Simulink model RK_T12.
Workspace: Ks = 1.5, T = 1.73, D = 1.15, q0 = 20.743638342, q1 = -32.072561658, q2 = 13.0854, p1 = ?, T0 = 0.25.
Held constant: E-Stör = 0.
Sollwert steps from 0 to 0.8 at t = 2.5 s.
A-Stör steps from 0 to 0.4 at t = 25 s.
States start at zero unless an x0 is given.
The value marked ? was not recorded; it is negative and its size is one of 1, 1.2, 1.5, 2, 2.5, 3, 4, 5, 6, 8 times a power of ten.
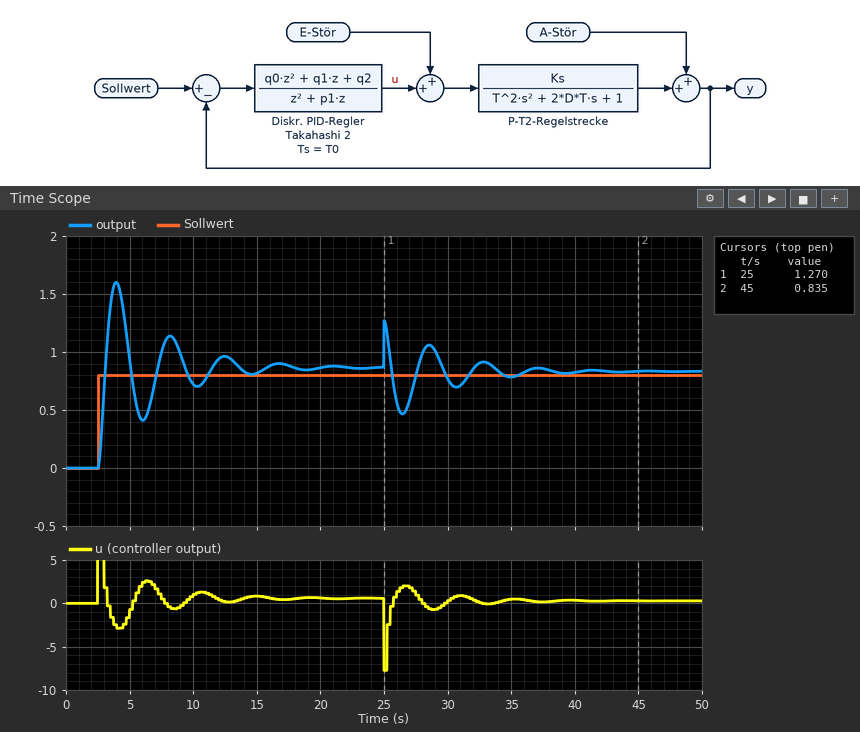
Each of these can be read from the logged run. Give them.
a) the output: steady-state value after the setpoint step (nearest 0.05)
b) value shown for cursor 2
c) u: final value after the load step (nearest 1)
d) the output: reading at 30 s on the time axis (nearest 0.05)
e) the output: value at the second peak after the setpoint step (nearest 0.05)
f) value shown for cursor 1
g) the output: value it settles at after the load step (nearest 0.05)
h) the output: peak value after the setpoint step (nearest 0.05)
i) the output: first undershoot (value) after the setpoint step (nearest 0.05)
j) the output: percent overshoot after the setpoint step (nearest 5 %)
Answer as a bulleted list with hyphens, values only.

- 0.85
- 0.835
- 0
- 0.75
- 1.15
- 1.270
- 0.85
- 1.60
- 0.40
- 85 %
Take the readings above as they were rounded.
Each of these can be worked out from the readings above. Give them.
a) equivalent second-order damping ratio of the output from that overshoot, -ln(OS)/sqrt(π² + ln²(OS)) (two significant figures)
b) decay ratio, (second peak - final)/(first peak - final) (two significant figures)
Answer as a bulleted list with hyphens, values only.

- 0.052
- 0.40
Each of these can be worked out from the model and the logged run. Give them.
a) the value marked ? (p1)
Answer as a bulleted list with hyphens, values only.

- -1.2
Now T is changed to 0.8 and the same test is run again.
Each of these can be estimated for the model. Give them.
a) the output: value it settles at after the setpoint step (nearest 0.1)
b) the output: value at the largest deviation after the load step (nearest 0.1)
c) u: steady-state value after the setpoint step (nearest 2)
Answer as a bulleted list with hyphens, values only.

- 0.9
- 0.5
- 0
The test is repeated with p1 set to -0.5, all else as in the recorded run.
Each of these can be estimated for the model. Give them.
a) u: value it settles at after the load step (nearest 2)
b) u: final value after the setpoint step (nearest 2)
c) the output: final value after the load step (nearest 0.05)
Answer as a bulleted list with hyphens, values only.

- 0
- 0
- 0.75
